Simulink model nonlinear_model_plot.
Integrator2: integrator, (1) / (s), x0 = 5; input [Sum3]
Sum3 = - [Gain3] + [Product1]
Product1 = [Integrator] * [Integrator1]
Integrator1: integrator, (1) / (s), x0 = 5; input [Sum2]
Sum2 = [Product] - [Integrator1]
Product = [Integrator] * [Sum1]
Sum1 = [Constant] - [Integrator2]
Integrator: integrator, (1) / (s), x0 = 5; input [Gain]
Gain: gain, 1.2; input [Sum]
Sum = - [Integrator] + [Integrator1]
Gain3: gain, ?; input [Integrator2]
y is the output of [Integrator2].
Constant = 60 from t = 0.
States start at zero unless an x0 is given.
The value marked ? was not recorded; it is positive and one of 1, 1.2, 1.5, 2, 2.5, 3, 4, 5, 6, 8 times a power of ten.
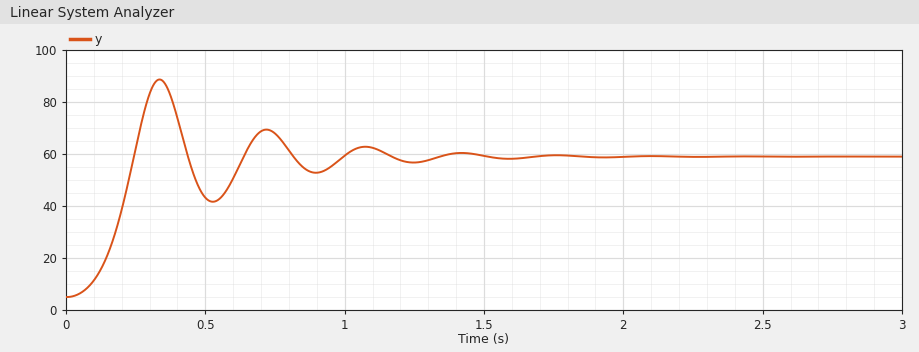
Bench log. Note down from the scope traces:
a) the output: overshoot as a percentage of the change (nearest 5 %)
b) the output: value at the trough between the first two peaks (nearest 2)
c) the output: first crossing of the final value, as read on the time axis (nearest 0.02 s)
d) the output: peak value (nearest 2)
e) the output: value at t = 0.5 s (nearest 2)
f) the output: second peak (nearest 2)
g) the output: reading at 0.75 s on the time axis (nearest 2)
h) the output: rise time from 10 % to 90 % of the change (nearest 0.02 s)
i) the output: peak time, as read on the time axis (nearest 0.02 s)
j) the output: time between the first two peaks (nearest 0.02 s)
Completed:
55 %
42
0.24 s
88
44
70
68
0.14 s
0.34 s
0.38 s
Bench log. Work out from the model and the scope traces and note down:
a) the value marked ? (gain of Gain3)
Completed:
6
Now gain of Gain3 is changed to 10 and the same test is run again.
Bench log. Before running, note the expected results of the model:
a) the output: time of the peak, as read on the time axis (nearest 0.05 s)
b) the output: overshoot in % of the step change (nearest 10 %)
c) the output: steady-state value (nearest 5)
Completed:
0.35 s
40 %
60
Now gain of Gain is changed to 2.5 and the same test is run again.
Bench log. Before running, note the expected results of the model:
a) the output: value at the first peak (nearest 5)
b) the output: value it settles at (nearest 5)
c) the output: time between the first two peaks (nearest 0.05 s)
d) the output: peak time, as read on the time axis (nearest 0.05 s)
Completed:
95
60
0.35 s
0.25 s
